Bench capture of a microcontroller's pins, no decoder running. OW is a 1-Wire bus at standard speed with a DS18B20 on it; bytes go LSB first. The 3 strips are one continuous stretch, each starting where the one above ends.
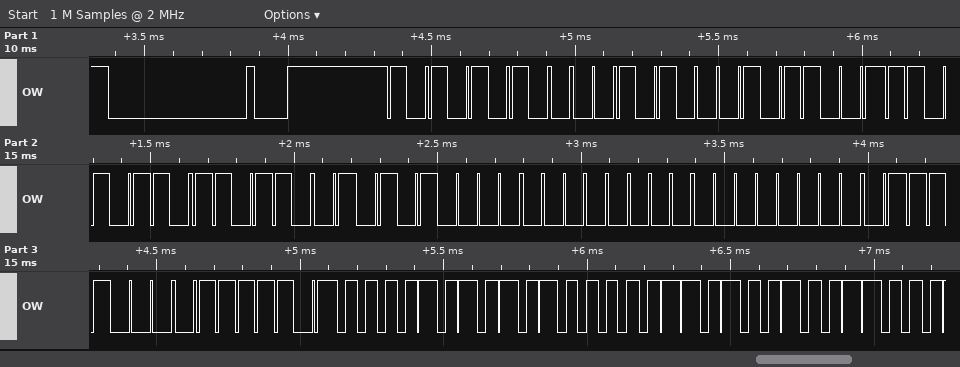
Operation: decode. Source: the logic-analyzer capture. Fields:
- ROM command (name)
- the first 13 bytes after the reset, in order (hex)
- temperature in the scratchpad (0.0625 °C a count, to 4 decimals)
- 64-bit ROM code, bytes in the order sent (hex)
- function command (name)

Match ROM
55 28 9A 6B 9B 0A 00 00 1E BE 50 05 4B
85.0000 °C
28 9A 6B 9B 0A 00 00 1E
Read Scratchpad
